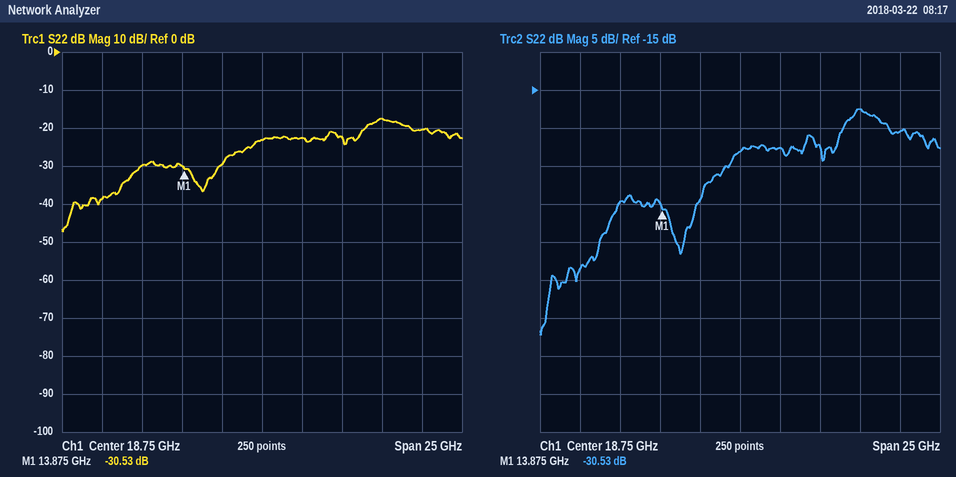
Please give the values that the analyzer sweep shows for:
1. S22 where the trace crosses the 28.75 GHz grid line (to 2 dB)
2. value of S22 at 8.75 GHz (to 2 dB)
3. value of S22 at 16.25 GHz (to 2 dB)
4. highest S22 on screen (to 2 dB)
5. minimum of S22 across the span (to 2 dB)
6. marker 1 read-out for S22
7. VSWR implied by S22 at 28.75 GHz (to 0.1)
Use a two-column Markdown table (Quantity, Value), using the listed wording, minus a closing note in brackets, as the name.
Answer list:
| Quantity | Value |
|---|---|
| S22 where the trace crosses the 28.75 GHz grid line | -20 dB |
| value of S22 at 8.75 GHz | -38 dB |
| value of S22 at 16.25 GHz | -30 dB |
| highest S22 on screen | -18 dB |
| minimum of S22 across the span | -48 dB |
| marker 1 read-out for S22 | -30.53 dB |
| VSWR implied by S22 at 28.75 GHz | 1.2 |
